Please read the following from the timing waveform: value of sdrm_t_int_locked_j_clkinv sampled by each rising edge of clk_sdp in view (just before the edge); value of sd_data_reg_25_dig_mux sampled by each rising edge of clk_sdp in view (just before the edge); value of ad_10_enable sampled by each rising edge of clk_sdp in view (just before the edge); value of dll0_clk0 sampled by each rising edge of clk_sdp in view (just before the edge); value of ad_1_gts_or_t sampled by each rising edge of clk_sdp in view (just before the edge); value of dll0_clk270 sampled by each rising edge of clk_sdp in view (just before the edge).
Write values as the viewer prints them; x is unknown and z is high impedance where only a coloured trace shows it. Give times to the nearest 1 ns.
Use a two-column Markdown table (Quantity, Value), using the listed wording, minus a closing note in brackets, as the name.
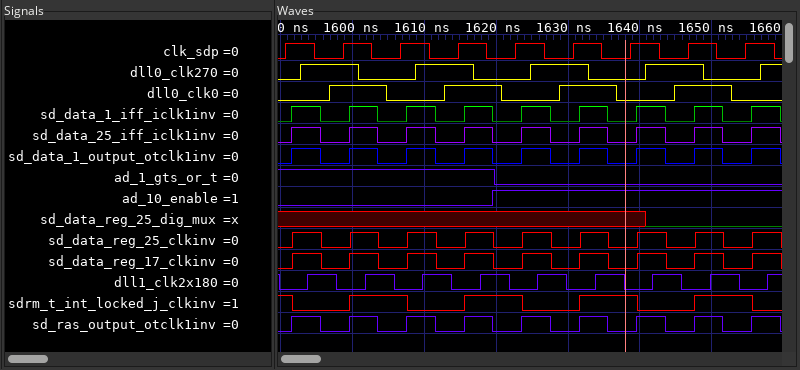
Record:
| Quantity | Value |
|---|---|
| value of sdrm_t_int_locked_j_clkinv sampled by each rising edge of clk_sdp in view | 1 0 1 0 1 0 1 0 1 |
| value of sd_data_reg_25_dig_mux sampled by each rising edge of clk_sdp in view | x x x x x x x 0 0 |
| value of ad_10_enable sampled by each rising edge of clk_sdp in view | 0 0 0 0 1 1 1 1 1 |
| value of dll0_clk0 sampled by each rising edge of clk_sdp in view | 0 1 0 1 0 1 0 1 0 |
| value of ad_1_gts_or_t sampled by each rising edge of clk_sdp in view | 1 1 1 1 0 0 0 0 0 |
| value of dll0_clk270 sampled by each rising edge of clk_sdp in view | 0 1 0 1 0 1 0 1 0 |
